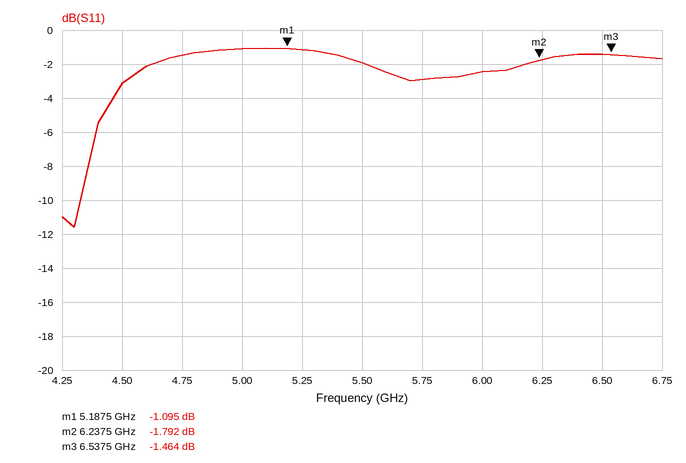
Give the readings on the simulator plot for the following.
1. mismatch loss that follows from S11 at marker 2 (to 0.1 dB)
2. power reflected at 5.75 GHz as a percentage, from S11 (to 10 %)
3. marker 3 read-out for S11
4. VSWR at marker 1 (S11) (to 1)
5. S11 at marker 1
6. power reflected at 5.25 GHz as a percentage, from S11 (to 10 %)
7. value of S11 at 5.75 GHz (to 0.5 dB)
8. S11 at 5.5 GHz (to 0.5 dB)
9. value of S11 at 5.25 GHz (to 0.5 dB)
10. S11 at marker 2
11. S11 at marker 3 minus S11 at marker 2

4.7 dB
50 %
-1.464 dB
16
-1.095 dB
80 %
-3.0 dB
-2.0 dB
-1.0 dB
-1.792 dB
0.328 dB
